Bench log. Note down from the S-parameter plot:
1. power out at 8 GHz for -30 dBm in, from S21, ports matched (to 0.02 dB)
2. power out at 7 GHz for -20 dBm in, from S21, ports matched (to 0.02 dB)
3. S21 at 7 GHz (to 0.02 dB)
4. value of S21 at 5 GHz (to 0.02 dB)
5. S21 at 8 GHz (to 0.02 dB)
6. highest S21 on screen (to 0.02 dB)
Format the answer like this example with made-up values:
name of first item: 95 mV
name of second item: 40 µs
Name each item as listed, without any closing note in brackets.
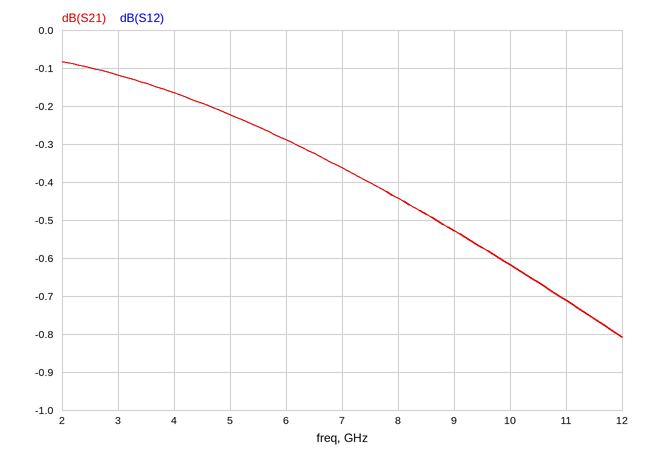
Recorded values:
power out at 8 GHz for -30 dBm in, from S21, ports matched: -30.44 dBm
power out at 7 GHz for -20 dBm in, from S21, ports matched: -20.36 dBm
S21 at 7 GHz: -0.36 dB
value of S21 at 5 GHz: -0.22 dB
S21 at 8 GHz: -0.44 dB
highest S21 on screen: -0.08 dB
